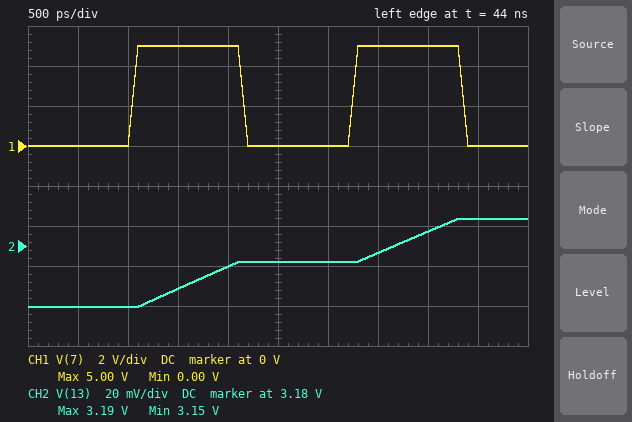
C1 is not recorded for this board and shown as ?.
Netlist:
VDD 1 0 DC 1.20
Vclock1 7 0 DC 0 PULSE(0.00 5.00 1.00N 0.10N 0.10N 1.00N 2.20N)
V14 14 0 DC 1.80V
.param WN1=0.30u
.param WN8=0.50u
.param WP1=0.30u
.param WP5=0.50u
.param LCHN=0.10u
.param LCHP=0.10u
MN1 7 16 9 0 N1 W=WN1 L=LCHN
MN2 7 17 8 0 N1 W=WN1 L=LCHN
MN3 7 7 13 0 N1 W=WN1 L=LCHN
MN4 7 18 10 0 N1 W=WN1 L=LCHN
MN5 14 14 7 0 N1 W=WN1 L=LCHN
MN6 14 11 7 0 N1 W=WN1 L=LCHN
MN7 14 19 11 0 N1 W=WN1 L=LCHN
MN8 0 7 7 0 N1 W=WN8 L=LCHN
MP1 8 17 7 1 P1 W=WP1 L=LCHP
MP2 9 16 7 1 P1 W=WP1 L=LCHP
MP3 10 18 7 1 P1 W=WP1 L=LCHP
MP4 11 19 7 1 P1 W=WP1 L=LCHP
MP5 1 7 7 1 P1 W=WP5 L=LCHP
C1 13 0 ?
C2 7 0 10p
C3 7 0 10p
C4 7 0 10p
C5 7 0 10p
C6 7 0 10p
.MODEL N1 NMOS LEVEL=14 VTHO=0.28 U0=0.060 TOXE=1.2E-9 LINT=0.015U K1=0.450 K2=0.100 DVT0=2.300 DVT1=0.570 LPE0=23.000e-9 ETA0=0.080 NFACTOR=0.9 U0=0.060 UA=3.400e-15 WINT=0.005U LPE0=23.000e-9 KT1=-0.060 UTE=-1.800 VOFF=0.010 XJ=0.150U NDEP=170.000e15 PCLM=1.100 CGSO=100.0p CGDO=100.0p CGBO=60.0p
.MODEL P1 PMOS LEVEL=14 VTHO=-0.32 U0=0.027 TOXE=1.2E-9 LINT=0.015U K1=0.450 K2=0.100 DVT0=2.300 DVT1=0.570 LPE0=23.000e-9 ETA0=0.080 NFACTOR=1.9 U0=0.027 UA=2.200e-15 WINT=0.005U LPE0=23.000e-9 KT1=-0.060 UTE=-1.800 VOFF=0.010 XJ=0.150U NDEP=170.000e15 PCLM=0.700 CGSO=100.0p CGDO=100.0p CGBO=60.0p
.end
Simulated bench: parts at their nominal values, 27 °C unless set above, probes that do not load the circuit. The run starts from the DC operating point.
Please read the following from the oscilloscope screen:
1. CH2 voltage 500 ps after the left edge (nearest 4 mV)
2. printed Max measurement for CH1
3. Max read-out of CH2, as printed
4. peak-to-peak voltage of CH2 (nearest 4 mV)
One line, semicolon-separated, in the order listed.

3.148 V; 5.00 V; 3.19 V; 44 mV
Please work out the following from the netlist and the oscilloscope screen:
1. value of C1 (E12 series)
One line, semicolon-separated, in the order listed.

27 pF
